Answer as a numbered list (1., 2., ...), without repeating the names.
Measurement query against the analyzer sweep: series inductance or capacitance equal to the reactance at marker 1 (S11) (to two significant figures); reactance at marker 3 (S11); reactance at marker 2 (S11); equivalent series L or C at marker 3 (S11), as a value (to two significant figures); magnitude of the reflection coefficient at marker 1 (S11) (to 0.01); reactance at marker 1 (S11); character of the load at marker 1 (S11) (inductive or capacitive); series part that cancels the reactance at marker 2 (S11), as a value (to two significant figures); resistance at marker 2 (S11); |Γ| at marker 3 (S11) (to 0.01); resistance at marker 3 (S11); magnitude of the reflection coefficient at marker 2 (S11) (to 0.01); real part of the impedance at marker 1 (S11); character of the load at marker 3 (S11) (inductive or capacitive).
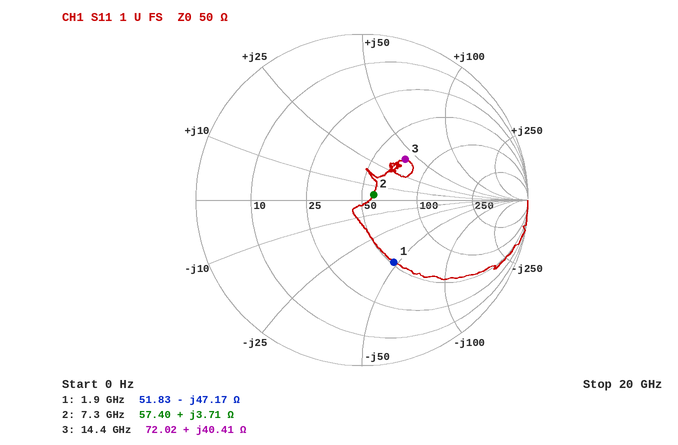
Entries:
1. 1.8 pF
2. +40.41 Ω
3. +3.71 Ω
4. 450 pH
5. 0.42
6. -47.17 Ω
7. capacitive
8. 5.9 pF
9. 57.40 Ω
10. 0.36
11. 72.02 Ω
12. 0.08
13. 51.83 Ω
14. inductive
